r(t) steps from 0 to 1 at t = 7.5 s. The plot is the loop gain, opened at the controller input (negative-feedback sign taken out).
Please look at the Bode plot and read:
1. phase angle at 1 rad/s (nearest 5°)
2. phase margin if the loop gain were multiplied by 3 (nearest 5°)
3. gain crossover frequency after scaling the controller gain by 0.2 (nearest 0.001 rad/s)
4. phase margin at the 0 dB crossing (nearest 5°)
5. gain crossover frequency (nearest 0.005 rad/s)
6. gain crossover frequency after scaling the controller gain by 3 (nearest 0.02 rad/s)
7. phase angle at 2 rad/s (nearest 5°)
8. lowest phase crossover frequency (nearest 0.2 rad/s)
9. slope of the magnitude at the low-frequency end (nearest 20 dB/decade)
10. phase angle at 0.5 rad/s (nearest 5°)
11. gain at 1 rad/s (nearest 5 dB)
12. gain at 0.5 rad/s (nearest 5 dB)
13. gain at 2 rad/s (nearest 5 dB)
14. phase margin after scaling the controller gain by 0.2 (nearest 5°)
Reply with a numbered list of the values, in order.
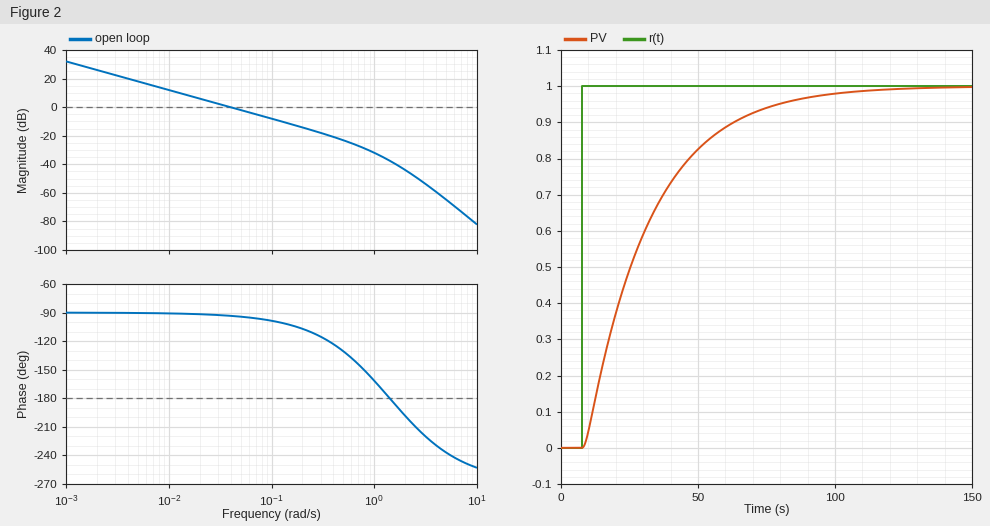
1. -160°
2. 80°
3. 0.008 rad/s
4. 85°
5. 0.040 rad/s
6. 0.12 rad/s
7. -200°
8. 1.4 rad/s
9. -20 dB/decade
10. -130°
11. -30 dB
12. -25 dB
13. -45 dB
14. 90°
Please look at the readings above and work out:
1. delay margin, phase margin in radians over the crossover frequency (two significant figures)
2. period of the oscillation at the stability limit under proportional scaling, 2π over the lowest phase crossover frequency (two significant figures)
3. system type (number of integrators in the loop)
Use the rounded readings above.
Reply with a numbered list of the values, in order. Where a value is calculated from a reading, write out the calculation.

1. 85 × π / 180 / 0.04 = 37 s
2. 2π / 1.4 = 4.5 s
3. 1
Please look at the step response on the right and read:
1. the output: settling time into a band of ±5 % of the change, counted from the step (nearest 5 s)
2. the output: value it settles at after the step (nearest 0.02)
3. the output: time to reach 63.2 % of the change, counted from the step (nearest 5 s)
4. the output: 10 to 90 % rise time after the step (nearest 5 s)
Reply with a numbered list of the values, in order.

1. 70 s
2. 1.00
3. 25 s
4. 50 s
